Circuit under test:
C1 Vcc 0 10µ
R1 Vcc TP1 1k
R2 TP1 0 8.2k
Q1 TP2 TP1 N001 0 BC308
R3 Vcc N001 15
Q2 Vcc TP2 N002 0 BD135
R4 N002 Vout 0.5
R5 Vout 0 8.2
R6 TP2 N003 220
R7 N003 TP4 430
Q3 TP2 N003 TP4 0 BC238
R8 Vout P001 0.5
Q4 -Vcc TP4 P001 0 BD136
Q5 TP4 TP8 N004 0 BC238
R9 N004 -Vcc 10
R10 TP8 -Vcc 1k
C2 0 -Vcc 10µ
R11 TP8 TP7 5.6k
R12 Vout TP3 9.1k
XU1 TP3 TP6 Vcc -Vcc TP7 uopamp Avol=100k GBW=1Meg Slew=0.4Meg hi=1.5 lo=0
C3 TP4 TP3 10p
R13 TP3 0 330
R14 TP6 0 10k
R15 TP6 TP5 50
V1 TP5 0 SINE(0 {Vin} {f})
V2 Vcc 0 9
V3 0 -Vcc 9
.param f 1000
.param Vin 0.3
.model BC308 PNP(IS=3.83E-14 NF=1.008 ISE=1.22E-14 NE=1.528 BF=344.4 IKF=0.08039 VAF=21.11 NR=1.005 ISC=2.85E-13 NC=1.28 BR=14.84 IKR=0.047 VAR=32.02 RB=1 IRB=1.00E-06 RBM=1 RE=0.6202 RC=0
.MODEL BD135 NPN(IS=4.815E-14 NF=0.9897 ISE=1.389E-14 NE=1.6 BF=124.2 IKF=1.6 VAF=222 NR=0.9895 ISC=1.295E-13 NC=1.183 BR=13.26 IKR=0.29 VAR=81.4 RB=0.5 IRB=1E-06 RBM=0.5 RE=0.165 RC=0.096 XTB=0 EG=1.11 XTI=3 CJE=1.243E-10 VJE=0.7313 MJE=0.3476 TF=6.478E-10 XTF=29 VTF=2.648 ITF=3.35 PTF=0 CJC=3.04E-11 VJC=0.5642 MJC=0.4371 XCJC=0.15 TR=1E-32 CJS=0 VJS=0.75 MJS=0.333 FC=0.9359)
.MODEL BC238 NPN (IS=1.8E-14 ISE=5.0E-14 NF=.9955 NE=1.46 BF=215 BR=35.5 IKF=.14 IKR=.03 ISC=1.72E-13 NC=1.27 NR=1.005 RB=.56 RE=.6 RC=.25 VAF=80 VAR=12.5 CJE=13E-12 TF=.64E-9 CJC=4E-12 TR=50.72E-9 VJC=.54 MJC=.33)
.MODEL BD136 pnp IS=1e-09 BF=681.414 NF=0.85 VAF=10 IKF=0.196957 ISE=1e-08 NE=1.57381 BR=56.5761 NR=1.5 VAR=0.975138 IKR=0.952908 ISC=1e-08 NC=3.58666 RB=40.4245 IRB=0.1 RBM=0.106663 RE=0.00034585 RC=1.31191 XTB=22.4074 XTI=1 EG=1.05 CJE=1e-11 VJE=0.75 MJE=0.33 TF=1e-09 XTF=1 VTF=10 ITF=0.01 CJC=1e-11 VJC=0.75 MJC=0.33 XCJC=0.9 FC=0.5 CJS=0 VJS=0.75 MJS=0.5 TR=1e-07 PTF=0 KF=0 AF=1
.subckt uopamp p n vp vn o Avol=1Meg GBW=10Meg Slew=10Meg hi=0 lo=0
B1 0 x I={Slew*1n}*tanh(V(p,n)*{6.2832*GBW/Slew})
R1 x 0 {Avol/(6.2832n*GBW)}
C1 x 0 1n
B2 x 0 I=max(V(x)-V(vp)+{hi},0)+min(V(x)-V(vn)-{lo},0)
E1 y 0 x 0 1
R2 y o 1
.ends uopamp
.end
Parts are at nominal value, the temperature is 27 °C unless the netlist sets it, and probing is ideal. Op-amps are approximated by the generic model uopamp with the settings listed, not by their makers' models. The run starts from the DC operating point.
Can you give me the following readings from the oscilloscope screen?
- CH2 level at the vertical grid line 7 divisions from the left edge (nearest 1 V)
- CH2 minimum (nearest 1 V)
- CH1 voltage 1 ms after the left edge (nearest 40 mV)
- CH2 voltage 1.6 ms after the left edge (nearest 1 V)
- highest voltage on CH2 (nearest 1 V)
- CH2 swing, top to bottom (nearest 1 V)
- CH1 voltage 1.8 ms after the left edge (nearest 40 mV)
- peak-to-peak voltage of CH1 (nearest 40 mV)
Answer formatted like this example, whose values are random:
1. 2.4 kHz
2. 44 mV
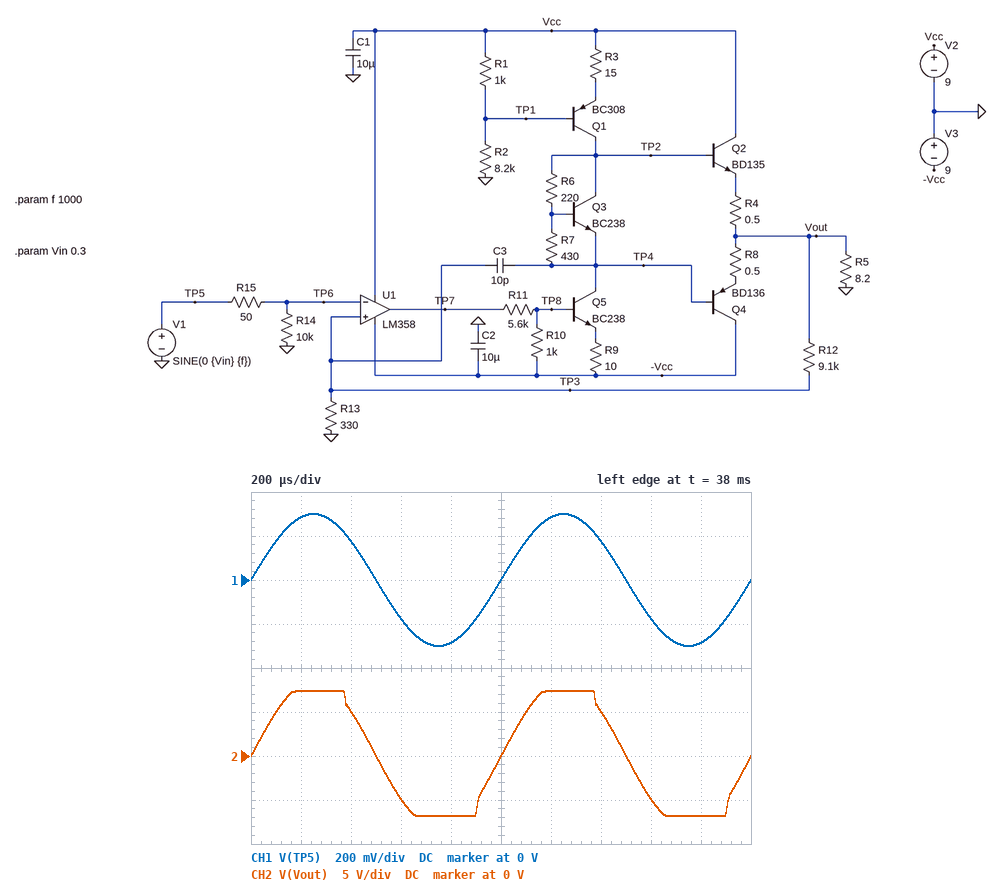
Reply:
1. 5 V
2. -7 V
3. 0 V
4. -5 V
5. 7 V
6. 14 V
7. -280 mV
8. 600 mV
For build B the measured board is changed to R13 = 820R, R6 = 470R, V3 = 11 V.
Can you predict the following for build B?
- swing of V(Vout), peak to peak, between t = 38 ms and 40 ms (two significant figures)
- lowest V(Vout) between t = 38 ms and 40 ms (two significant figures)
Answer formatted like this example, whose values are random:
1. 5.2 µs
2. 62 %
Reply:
1. 7.2 V
2. -3.6 V
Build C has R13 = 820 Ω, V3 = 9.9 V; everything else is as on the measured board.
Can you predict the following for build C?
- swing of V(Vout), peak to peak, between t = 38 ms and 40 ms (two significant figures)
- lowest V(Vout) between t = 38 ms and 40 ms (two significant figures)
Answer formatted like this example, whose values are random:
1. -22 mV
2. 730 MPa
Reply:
1. 7.2 V
2. -3.6 V
